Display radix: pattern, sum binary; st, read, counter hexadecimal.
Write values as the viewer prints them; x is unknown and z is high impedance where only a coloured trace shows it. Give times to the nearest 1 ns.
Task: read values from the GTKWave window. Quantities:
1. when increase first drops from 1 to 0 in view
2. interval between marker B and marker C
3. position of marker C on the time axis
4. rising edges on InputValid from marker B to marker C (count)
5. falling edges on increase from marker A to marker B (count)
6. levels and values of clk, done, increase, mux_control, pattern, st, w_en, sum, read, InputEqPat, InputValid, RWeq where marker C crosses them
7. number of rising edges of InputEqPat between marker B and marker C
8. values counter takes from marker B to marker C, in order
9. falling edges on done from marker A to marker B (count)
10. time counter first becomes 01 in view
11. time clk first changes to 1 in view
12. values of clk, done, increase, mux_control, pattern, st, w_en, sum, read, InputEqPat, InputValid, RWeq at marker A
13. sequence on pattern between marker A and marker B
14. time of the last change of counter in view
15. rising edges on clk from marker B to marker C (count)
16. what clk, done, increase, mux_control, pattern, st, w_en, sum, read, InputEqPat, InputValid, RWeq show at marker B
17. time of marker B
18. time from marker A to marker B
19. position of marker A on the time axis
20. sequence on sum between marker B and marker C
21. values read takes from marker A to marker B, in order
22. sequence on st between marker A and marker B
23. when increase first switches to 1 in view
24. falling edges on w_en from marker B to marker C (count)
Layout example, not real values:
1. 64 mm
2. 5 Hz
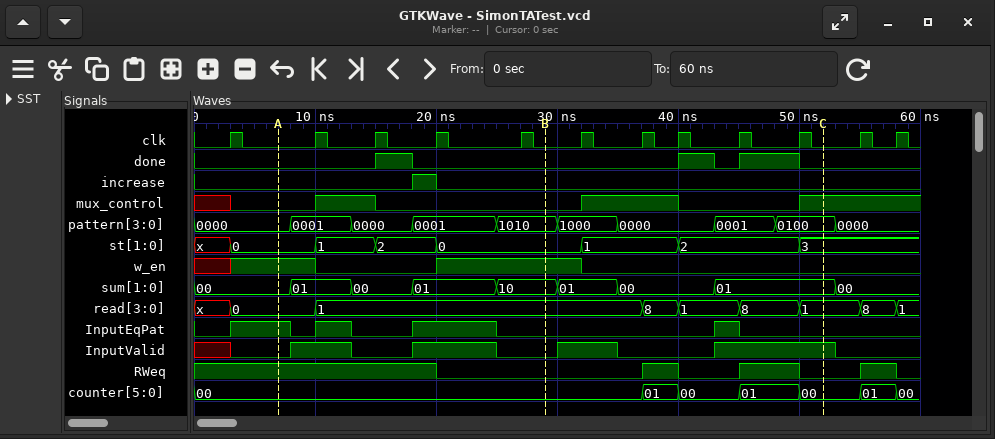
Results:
1. 20 ns
2. 23 ns
3. 52 ns
4. 2
5. 1
6. clk=0, done=0, increase=0, mux_control=1, pattern=0100, st=3, w_en=0, sum=01, read=1, InputEqPat=0, InputValid=1, RWeq=0
7. 1
8. 00, 01, 00, 01, 00
9. 1
10. 37 ns
11. 3 ns
12. clk=0, done=0, increase=0, mux_control=0, pattern=0000, st=0, w_en=1, sum=00, read=0, InputEqPat=1, InputValid=0, RWeq=1
13. 0000, 0001, 0000, 0001, 1010
14. 58 ns
15. 5
16. clk=0, done=0, increase=0, mux_control=0, pattern=1010, st=0, w_en=1, sum=10, read=1, InputEqPat=0, InputValid=0, RWeq=0
17. 29 ns
18. 22 ns
19. 7 ns
20. 10, 01, 00, 01
21. 0, 1
22. 0, 1, 2, 0
23. 18 ns
24. 1
